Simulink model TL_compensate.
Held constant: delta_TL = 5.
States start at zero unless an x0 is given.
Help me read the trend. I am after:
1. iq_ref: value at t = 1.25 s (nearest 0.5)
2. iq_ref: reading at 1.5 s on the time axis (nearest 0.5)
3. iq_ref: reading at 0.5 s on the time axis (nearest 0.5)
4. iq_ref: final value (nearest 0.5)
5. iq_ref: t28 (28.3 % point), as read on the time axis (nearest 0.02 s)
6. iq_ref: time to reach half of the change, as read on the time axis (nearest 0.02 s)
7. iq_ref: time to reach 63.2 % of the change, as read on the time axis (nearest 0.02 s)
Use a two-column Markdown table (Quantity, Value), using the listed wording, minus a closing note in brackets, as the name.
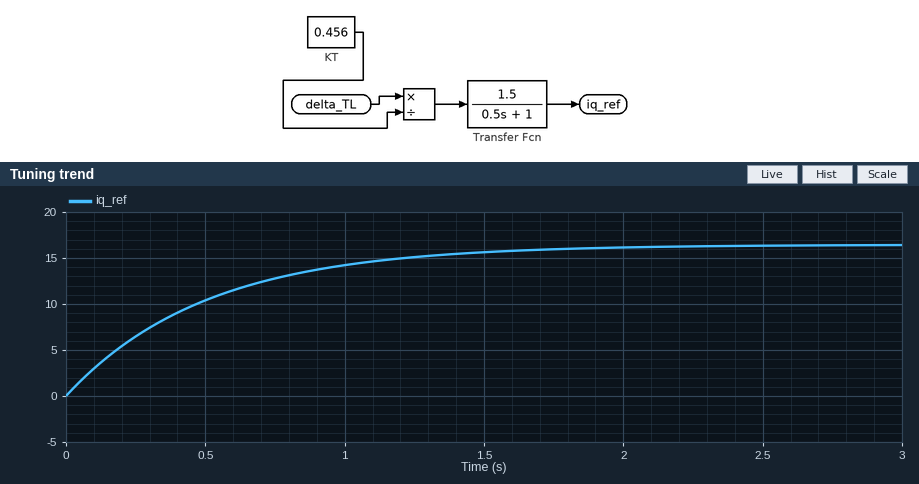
| Quantity | Value |
|---|---|
| iq_ref: value at t = 1.25 s | 15.0 |
| iq_ref: reading at 1.5 s on the time axis | 15.5 |
| iq_ref: reading at 0.5 s on the time axis | 10.5 |
| iq_ref: final value | 16.5 |
| iq_ref: t28 (28.3 % point), as read on the time axis | 0.16 s |
| iq_ref: time to reach half of the change, as read on the time axis | 0.34 s |
| iq_ref: time to reach 63.2 % of the change, as read on the time axis | 0.50 s |
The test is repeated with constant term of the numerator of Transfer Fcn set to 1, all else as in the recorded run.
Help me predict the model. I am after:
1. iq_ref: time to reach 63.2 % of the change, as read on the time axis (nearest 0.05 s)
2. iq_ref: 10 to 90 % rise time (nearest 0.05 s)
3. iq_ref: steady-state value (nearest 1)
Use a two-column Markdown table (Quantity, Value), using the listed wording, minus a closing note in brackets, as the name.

| Quantity | Value |
|---|---|
| iq_ref: time to reach 63.2 % of the change, as read on the time axis | 0.50 s |
| iq_ref: 10 to 90 % rise time | 1.10 s |
| iq_ref: steady-state value | 11 |
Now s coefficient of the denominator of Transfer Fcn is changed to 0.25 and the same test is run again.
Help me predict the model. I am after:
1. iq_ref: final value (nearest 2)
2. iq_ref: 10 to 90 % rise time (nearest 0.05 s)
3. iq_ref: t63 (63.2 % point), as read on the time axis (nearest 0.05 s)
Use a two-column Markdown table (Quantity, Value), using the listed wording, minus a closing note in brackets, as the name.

| Quantity | Value |
|---|---|
| iq_ref: final value | 16 |
| iq_ref: 10 to 90 % rise time | 0.55 s |
| iq_ref: t63 (63.2 % point), as read on the time axis | 0.25 s |
